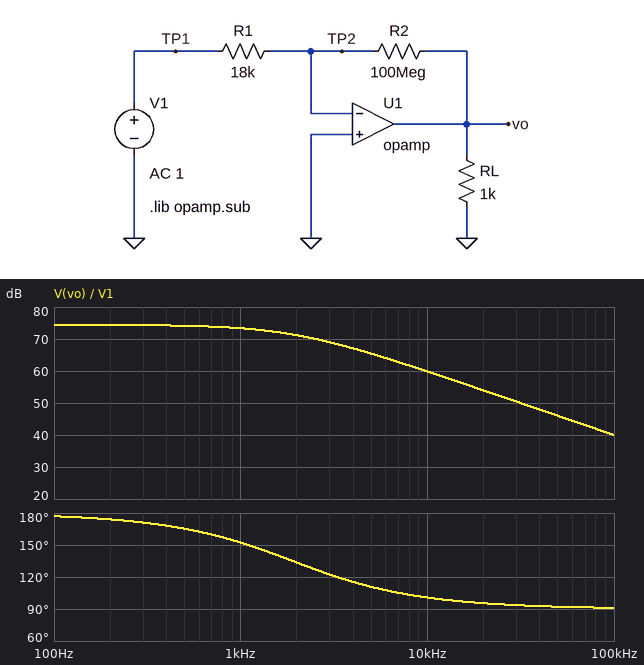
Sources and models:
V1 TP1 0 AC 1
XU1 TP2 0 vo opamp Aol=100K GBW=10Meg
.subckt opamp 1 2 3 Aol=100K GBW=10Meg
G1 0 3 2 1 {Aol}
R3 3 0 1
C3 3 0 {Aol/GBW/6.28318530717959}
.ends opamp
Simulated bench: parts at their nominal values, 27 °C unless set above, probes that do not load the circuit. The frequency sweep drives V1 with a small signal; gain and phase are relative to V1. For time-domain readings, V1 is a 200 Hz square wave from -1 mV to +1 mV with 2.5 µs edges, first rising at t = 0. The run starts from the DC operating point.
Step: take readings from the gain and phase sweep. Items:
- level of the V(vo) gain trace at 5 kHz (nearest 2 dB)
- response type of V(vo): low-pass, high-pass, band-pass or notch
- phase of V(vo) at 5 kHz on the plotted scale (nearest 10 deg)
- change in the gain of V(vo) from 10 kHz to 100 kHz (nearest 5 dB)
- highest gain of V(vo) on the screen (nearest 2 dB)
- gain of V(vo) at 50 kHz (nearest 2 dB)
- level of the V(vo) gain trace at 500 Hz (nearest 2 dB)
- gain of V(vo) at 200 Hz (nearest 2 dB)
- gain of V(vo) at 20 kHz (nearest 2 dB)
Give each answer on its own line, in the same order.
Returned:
66 dB
low-pass
110 deg
-20 dB
74 dB
46 dB
74 dB
74 dB
54 dB
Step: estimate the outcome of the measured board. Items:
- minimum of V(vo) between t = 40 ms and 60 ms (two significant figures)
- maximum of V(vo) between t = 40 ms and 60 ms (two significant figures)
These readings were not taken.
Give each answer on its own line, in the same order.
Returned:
-5.3 V
5.3 V
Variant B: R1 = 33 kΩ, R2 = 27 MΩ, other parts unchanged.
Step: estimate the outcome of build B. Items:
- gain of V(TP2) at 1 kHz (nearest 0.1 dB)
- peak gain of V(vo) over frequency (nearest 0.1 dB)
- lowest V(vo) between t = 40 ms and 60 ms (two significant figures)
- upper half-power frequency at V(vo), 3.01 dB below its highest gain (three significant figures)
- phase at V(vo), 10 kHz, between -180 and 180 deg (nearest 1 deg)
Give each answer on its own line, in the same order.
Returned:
-21.8 dB
58.2 dB
-810 mV
12.3 kHz
141 deg
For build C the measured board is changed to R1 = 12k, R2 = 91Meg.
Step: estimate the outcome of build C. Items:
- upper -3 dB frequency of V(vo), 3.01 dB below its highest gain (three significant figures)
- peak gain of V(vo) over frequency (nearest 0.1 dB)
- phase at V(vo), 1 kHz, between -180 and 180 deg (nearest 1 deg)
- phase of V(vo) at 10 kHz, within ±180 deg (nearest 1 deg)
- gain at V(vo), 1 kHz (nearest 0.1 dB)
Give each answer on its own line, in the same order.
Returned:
1.42 kHz
77.0 dB
145 deg
98 deg
75.2 dB
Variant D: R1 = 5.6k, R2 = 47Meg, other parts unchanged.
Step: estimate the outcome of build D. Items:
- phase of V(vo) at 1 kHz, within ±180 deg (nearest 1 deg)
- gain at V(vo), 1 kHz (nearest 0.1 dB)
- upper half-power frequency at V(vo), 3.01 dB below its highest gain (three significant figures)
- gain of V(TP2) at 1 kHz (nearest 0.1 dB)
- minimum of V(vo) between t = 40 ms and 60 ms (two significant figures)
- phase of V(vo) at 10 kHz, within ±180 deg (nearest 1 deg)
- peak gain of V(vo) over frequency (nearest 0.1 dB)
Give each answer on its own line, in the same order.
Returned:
142 deg
75.7 dB
1.29 kHz
-4.2 dB
-7.7 V
97 deg
77.8 dB
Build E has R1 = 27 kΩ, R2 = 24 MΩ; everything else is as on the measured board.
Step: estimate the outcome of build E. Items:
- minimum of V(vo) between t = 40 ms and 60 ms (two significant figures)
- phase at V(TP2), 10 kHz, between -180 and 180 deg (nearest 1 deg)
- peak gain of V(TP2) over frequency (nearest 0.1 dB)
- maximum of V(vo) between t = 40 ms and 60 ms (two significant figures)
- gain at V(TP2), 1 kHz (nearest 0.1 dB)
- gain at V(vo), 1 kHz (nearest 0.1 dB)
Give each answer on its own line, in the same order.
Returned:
-880 mV
48 deg
0 dB
880 mV
-21.1 dB
58.9 dB
